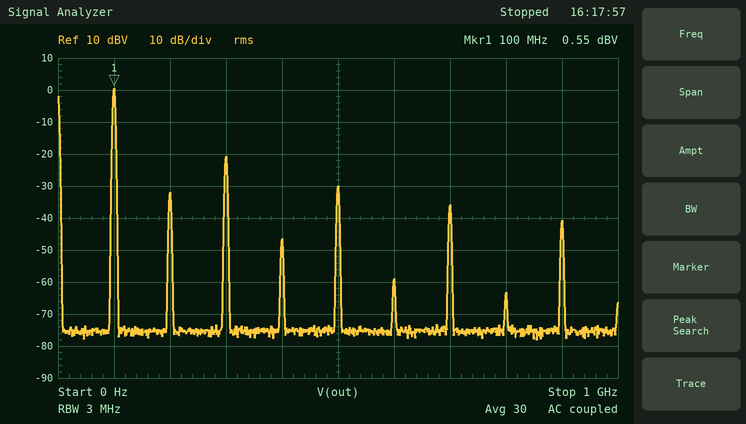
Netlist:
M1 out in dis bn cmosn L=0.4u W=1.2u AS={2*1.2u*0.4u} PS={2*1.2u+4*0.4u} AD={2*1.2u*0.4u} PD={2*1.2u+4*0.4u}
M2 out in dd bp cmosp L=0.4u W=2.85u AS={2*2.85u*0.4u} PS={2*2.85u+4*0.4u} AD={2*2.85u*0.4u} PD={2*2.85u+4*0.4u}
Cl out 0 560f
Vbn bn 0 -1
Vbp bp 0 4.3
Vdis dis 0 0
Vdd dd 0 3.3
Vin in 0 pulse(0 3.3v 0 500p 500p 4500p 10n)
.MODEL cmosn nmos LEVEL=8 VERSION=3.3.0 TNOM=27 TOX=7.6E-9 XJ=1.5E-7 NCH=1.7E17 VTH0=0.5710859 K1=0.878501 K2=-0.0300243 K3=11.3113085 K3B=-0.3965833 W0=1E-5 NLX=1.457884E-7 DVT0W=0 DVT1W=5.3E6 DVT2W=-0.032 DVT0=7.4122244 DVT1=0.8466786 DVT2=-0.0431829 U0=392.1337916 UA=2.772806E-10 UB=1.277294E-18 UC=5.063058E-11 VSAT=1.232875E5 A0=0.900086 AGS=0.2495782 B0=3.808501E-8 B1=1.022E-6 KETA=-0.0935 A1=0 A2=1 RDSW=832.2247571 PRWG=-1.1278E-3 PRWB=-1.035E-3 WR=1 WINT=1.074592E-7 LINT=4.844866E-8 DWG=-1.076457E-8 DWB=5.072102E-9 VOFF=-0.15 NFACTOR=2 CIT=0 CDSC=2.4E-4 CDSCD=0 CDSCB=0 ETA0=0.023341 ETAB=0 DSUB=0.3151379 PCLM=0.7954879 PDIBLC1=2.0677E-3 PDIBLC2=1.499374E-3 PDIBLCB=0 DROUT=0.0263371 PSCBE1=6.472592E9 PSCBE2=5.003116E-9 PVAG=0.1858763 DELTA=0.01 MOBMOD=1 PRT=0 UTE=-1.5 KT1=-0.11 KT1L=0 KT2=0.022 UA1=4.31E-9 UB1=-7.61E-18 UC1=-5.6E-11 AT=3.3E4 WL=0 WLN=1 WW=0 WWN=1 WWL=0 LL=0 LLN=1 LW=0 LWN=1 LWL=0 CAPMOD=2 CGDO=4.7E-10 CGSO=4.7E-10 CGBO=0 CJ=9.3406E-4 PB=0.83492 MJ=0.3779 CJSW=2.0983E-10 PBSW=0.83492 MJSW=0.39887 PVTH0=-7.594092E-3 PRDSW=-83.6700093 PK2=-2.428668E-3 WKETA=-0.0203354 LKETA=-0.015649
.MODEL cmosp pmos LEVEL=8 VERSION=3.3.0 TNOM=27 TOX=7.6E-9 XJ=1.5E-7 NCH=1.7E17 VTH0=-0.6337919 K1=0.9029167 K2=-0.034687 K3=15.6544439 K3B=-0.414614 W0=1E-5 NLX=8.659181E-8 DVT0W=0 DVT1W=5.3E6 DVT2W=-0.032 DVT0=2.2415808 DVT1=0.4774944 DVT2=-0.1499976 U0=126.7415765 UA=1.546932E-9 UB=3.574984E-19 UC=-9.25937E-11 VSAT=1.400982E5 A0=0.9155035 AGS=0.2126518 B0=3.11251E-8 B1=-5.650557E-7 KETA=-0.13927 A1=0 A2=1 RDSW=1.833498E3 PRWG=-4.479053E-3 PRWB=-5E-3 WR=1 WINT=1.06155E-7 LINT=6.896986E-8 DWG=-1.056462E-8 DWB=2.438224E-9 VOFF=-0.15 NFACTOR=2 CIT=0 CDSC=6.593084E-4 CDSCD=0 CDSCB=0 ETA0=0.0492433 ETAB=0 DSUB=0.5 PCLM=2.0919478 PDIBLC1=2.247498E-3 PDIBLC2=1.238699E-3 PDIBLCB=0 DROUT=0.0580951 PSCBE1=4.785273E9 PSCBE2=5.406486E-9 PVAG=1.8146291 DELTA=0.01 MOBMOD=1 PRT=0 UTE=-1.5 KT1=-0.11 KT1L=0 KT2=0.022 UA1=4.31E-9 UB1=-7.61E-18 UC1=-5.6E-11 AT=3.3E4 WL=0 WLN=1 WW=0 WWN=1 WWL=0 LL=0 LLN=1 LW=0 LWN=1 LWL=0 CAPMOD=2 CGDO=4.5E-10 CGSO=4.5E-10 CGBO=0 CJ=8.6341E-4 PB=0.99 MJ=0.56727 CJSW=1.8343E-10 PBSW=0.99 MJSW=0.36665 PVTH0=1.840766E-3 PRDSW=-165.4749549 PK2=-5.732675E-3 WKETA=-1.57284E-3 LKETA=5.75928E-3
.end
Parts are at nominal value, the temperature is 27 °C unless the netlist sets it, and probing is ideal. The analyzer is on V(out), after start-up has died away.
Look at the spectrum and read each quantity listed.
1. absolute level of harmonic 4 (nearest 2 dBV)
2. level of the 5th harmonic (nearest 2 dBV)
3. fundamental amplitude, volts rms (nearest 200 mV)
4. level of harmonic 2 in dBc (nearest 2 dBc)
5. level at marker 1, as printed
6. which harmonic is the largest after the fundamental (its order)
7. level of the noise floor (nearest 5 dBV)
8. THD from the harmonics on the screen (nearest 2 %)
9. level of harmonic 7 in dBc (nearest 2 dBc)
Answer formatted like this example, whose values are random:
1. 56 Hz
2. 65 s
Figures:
1. -46 dBV
2. -30 dBV
3. 1.0 V
4. -32 dBc
5. 0.55 dBV
6. 3
7. -75 dBV
8. 10 %
9. -36 dBc
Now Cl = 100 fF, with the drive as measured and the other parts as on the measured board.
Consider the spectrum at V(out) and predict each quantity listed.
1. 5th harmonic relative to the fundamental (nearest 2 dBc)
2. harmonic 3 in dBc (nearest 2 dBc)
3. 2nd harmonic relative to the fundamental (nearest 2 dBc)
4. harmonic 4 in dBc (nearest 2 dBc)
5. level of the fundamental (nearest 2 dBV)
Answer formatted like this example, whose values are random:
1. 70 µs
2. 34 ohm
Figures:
1. -16 dBc
2. -10 dBc
3. -46 dBc
4. -44 dBc
5. 4 dBV
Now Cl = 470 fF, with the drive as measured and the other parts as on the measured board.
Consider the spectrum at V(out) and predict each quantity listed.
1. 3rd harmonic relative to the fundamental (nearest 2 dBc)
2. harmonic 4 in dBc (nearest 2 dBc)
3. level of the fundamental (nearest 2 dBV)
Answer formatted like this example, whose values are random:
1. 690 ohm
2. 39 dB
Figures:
1. -20 dBc
2. -44 dBc
3. 2 dBV
